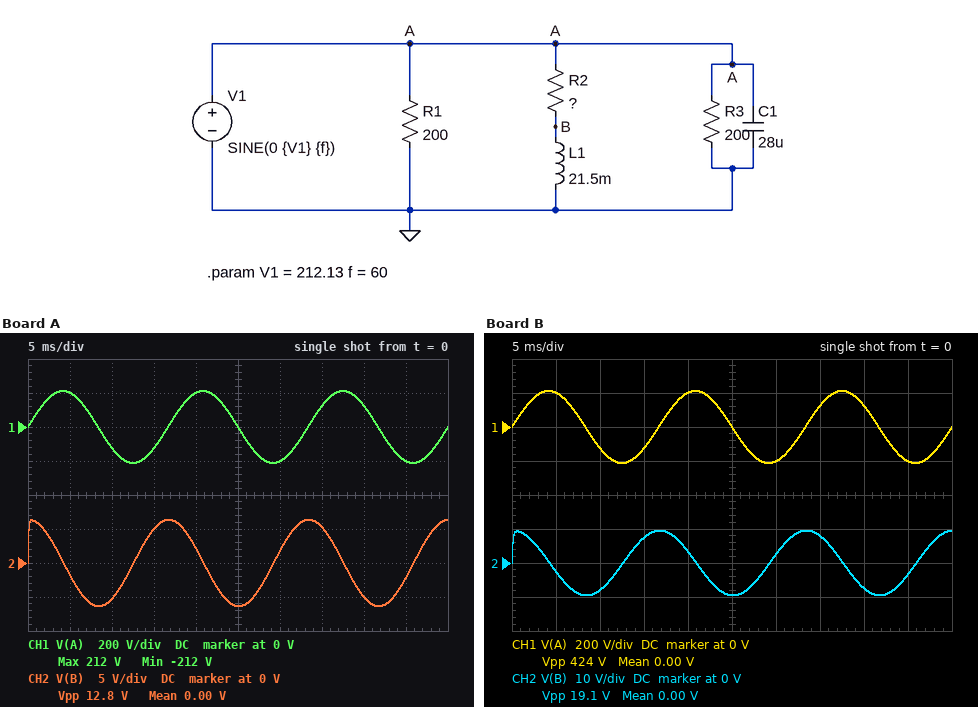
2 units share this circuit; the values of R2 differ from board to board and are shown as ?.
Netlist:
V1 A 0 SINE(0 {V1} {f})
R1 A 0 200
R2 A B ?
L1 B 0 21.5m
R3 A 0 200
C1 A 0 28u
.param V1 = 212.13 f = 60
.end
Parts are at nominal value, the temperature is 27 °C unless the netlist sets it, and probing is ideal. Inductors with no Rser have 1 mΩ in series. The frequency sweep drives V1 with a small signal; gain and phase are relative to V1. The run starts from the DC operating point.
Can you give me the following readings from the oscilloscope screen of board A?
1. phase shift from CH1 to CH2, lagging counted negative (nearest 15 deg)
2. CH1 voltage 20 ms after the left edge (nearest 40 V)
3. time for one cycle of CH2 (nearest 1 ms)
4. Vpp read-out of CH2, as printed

90 deg
200 V
17 ms
12.8 V
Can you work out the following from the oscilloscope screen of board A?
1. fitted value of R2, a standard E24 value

270 Ω
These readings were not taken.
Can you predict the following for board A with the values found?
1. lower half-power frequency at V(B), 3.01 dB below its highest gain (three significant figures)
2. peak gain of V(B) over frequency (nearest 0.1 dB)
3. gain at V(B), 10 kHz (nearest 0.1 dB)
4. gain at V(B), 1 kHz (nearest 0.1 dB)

2.00 kHz
0 dB
-0.2 dB
-7.0 dB
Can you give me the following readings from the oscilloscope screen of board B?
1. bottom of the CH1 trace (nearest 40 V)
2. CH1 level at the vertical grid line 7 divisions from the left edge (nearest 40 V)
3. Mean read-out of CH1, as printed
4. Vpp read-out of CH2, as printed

-200 V
120 V
0.00 V
19.1 V
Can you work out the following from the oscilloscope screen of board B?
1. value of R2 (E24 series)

180 Ω
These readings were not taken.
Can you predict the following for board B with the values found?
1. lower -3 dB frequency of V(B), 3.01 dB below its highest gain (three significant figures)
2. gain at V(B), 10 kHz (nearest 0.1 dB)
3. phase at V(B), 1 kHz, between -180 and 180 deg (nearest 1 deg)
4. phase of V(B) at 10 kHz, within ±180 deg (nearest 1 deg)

1.33 kHz
-0.1 dB
53 deg
8 deg
